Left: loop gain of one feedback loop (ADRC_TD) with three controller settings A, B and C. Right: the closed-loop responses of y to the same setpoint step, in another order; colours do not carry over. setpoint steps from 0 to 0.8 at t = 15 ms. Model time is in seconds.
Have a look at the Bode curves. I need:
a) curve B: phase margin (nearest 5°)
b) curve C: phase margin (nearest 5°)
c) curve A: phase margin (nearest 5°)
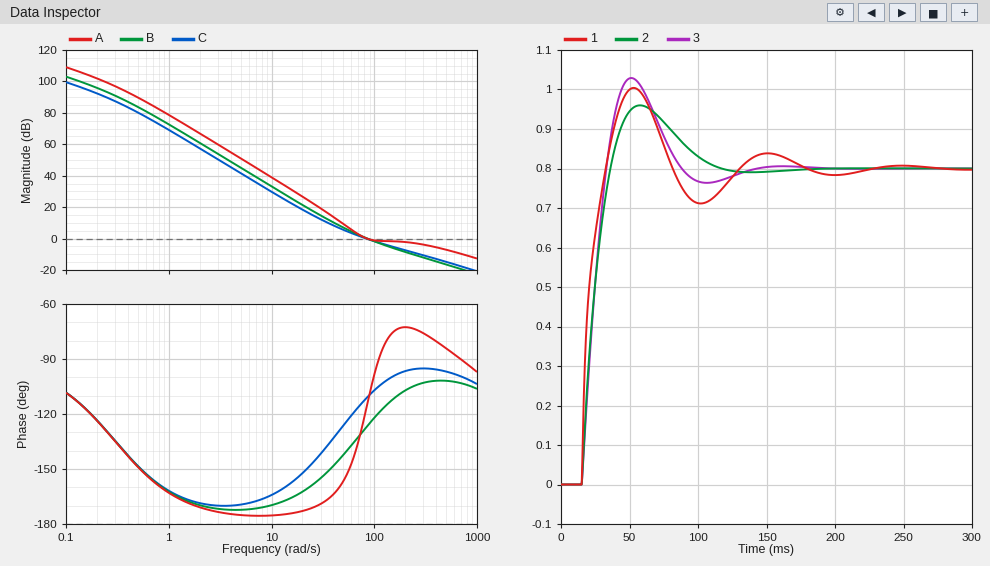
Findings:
55°
70°
65°
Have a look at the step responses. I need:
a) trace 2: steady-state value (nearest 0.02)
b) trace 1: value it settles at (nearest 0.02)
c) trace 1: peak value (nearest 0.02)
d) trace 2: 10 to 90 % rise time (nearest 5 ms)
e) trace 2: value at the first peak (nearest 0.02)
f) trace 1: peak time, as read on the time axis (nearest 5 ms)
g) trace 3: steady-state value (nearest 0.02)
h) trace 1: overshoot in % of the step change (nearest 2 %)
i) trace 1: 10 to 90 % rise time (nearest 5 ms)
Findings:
0.80
0.80
1.00
15 ms
0.96
55 ms
0.80
26 %
15 ms
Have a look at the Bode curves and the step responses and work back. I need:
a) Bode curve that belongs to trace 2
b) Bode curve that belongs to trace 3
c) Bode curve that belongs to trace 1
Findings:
C
B
A
